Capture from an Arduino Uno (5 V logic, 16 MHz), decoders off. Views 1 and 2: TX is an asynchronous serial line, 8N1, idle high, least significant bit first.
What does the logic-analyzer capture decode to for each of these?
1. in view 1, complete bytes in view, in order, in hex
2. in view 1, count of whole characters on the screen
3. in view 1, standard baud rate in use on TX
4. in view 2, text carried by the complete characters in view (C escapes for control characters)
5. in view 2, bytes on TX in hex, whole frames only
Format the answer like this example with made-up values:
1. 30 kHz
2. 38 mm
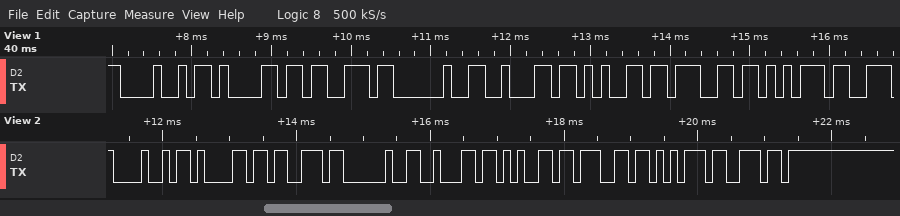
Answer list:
1. 48 61 73 20 62 65 67 75
2. 8
3. 9600 baud
4. "Has begun"
5. 48 61 73 20 62 65 67 75 6E
